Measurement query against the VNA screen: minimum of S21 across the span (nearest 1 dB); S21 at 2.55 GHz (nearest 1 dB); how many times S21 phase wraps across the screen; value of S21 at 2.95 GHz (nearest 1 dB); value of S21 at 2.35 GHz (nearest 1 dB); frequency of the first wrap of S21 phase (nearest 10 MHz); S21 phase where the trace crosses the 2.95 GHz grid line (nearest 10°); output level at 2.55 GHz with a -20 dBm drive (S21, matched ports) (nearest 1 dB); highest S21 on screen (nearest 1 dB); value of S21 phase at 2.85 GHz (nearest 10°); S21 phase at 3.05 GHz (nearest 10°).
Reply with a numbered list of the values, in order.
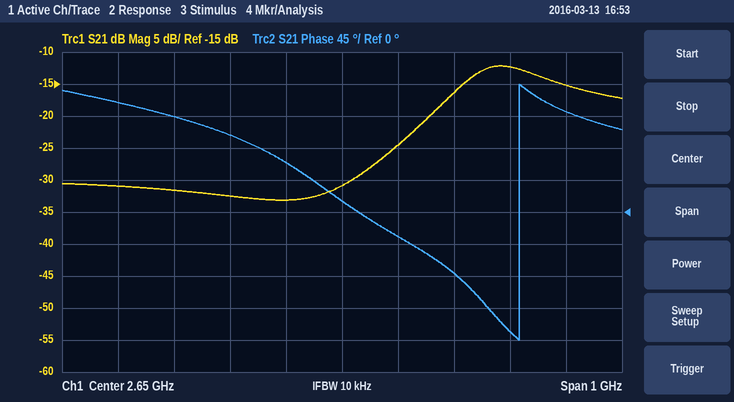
1. -33 dB
2. -33 dB
3. 1
4. -12 dB
5. -32 dB
6. 2.97 GHz
7. -170°
8. -53 dBm
9. -12 dB
10. -90°
11. 140°
